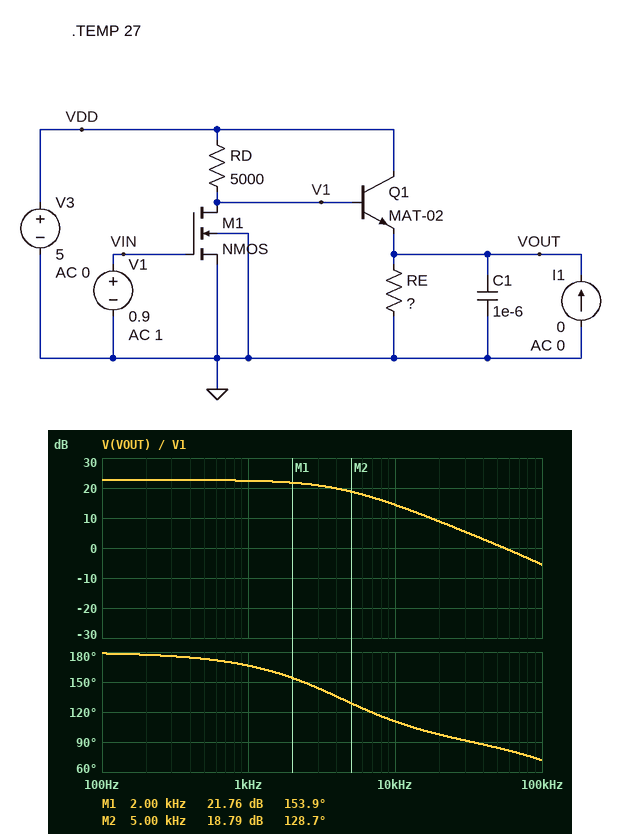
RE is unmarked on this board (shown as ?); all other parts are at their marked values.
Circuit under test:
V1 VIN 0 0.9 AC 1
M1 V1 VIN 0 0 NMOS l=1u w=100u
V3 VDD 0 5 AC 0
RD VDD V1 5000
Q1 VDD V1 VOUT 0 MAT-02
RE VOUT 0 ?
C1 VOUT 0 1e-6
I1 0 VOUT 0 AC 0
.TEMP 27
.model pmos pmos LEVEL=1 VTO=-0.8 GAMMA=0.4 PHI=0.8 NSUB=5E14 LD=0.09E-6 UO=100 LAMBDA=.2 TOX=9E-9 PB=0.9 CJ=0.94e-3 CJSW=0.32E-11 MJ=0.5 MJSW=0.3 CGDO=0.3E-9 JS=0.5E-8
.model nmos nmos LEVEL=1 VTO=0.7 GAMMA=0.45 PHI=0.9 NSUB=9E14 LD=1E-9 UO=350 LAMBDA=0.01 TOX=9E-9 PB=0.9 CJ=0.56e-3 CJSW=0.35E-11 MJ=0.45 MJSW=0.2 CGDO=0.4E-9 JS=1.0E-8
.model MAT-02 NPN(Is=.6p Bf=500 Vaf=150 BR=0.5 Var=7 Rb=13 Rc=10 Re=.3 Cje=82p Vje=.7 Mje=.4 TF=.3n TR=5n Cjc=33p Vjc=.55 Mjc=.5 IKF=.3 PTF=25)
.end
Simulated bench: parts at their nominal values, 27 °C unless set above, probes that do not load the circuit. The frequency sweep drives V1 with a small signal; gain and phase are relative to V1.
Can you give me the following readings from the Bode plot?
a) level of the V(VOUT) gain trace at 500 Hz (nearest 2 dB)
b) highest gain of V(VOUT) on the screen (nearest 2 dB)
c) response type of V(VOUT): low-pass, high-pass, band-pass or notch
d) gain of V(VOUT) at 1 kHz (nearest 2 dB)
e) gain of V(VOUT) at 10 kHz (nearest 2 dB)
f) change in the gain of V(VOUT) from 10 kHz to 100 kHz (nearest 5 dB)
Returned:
22 dB
22 dB
low-pass
22 dB
14 dB
-20 dB
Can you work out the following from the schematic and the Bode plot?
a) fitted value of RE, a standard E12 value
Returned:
3.3 kΩ
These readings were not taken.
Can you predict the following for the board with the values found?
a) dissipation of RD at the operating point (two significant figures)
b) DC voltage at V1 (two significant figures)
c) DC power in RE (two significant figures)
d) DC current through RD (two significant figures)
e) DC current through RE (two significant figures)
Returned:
390 µW
3.6 V
2.8 mW
280 µA
920 µA
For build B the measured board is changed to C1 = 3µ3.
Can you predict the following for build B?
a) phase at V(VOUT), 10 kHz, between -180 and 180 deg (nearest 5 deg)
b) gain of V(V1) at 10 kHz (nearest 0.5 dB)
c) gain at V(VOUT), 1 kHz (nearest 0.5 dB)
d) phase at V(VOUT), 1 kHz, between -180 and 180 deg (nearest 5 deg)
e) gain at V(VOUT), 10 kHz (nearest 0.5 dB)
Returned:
95 deg
20.0 dB
20.5 dB
140 deg
4.5 dB
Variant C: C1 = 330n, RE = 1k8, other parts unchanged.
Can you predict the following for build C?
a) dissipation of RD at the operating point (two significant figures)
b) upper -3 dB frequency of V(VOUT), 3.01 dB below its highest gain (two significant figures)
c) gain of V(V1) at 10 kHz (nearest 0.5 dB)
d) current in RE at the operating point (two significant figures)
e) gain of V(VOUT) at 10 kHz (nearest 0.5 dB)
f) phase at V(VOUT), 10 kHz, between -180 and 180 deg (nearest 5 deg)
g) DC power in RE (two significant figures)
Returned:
400 µW
19 kHz
22.0 dB
1.7 mA
21.5 dB
150 deg
5.1 mW
